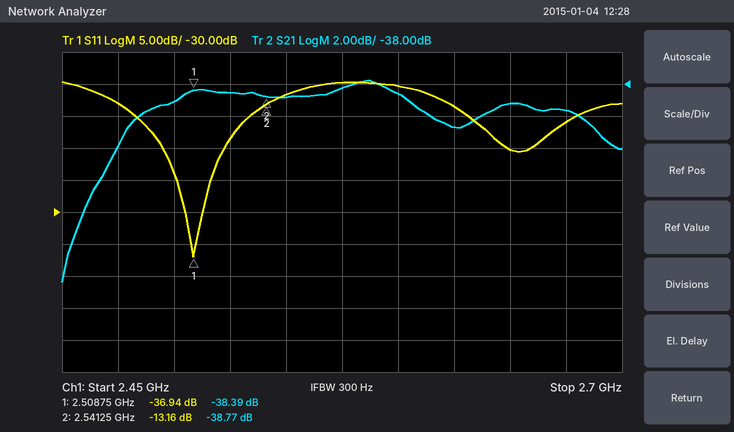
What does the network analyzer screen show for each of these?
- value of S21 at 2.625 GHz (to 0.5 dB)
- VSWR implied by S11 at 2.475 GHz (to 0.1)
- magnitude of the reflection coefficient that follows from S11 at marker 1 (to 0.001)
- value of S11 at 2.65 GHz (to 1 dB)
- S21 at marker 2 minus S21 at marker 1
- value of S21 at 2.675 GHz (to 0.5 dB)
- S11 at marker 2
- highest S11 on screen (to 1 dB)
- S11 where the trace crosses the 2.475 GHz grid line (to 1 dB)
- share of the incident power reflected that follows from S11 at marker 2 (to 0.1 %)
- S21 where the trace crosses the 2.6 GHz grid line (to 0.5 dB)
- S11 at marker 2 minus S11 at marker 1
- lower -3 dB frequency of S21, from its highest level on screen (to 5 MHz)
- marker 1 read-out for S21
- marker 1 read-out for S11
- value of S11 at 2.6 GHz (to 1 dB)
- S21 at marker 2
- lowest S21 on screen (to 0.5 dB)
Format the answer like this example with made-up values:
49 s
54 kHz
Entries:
-40.5 dB
1.6
0.014
-20 dB
-0.38 dB
-39.5 dB
-13.16 dB
-10 dB
-13 dB
4.8 %
-38.5 dB
23.78 dB
2.480 GHz
-38.39 dB
-36.94 dB
-10 dB
-38.77 dB
-50.5 dB
